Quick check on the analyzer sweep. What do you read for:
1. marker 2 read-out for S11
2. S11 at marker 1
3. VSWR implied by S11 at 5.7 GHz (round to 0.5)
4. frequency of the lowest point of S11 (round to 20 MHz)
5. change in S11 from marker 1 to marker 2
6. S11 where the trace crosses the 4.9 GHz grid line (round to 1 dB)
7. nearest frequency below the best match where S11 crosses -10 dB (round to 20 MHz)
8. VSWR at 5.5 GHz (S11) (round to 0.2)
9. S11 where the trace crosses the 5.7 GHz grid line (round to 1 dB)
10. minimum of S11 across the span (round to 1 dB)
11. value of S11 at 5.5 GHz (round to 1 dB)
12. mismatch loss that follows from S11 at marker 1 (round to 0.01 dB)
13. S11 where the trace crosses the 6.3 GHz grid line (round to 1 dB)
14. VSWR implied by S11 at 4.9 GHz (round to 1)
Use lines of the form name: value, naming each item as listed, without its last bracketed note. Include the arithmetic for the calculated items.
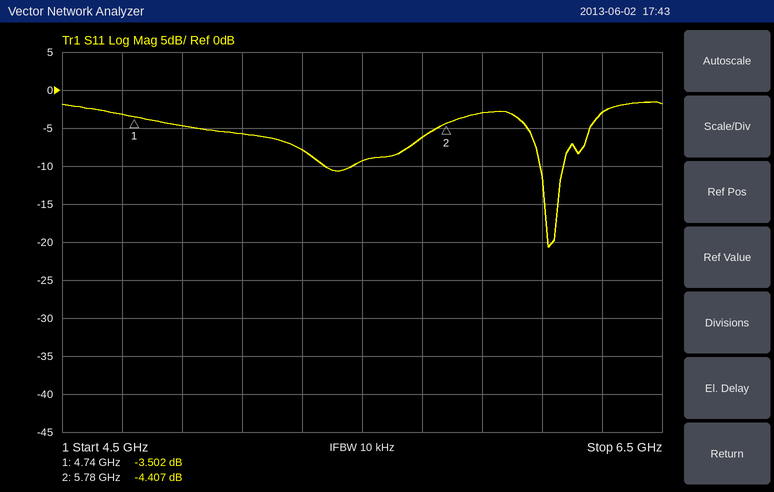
marker 2 read-out for S11: -4.407 dB
S11 at marker 1: -3.502 dB
VSWR implied by S11 at 5.7 GHz: |Γ| = 10^(-6/20) = 0.5012; VSWR = (1 + 0.5012)/(1 − 0.5012) ≈ 3.0
frequency of the lowest point of S11: 6.12 GHz
change in S11 from marker 1 to marker 2: -4.407 − (-3.502) = -0.905 dB
S11 where the trace crosses the 4.9 GHz grid line: -5 dB
nearest frequency below the best match where S11 crosses -10 dB: 6.10 GHz
VSWR at 5.5 GHz (S11): |Γ| = 10^(-9/20) = 0.3548; VSWR = (1 + 0.3548)/(1 − 0.3548) ≈ 2.10, so 2.0 to the nearest 0.2
S11 where the trace crosses the 5.7 GHz grid line: -6 dB
minimum of S11 across the span: -21 dB
value of S11 at 5.5 GHz: -9 dB
mismatch loss that follows from S11 at marker 1: −10 log10(1 − 10^(-3.502/10)) ≈ 2.57 dB
S11 where the trace crosses the 6.3 GHz grid line: -3 dB
VSWR implied by S11 at 4.9 GHz: |Γ| = 10^(-5/20) = 0.5623; VSWR = (1 + 0.5623)/(1 − 0.5623) ≈ 4
